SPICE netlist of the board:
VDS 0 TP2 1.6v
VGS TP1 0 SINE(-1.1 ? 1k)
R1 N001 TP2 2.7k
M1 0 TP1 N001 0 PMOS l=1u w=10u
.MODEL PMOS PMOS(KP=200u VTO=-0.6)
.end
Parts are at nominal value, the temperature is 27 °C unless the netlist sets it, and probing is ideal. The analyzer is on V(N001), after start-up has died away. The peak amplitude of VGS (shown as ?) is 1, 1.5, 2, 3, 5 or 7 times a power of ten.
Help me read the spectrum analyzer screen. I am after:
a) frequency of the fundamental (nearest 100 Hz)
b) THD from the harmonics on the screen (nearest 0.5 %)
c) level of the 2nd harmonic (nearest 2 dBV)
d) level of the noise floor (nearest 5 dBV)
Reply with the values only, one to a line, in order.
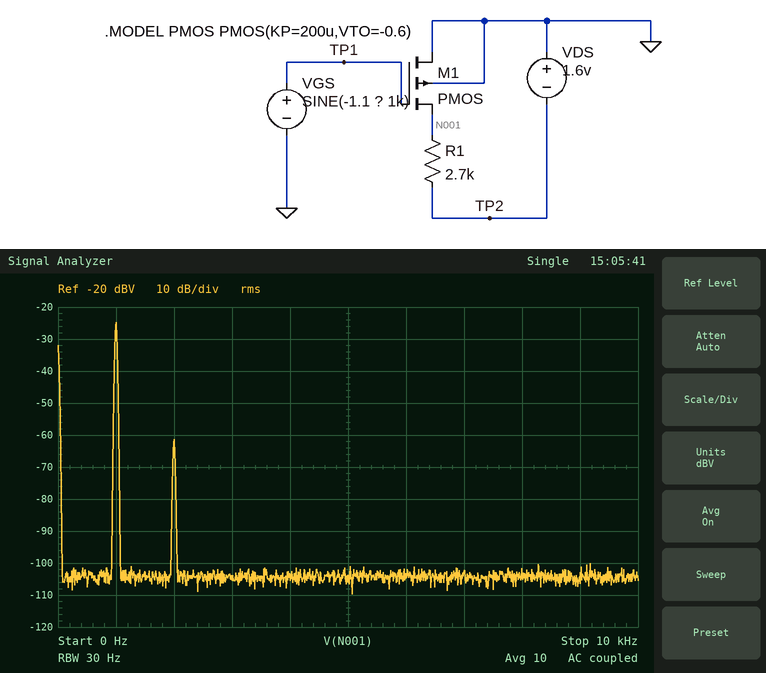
1.0 kHz
1.5 %
-62 dBV
-105 dBV
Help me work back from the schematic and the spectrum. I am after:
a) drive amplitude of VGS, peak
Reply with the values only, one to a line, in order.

30 mV
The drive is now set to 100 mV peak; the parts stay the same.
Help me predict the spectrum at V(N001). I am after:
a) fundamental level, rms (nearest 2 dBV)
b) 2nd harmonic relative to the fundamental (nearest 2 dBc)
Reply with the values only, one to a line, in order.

-14 dBV
-26 dBc
